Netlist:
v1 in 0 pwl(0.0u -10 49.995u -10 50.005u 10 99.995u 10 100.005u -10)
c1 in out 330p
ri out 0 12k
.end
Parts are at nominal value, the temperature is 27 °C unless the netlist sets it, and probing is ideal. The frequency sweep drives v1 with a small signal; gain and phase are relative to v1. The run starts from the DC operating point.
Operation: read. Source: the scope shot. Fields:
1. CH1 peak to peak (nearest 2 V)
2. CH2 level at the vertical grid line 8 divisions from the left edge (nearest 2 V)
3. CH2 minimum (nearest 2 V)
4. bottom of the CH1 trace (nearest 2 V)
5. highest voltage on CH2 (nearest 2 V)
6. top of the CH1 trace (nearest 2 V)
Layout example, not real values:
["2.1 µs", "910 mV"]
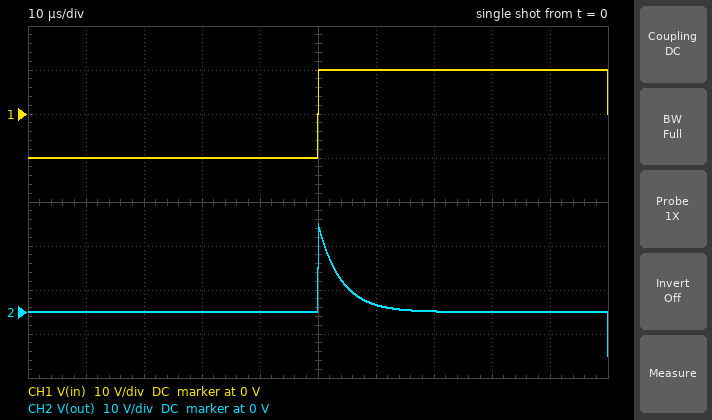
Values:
["20 V", "0 V", "-10 V", "-10 V", "20 V", "10 V"]
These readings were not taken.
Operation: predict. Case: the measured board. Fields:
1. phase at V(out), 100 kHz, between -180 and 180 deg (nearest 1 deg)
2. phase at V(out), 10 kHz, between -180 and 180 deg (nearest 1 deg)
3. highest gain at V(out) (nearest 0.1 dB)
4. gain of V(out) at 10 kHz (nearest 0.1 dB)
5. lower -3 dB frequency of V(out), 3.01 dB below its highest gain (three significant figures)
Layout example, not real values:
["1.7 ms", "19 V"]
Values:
["22 deg", "76 deg", "0 dB", "-12.3 dB", "40.2 kHz"]
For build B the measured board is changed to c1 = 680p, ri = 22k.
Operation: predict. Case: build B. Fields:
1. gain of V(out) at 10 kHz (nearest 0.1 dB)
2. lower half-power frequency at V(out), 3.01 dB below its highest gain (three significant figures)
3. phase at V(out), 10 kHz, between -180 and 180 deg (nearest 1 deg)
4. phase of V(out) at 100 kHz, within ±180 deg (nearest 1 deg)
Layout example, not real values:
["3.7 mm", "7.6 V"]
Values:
["-3.3 dB", "10.6 kHz", "47 deg", "6 deg"]
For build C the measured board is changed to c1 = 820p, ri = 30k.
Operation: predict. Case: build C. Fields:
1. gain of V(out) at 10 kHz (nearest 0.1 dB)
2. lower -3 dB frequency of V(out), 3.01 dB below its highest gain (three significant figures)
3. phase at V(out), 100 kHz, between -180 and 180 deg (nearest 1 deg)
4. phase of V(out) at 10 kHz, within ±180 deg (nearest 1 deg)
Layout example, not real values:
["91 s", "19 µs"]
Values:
["-1.5 dB", "6.47 kHz", "4 deg", "33 deg"]
